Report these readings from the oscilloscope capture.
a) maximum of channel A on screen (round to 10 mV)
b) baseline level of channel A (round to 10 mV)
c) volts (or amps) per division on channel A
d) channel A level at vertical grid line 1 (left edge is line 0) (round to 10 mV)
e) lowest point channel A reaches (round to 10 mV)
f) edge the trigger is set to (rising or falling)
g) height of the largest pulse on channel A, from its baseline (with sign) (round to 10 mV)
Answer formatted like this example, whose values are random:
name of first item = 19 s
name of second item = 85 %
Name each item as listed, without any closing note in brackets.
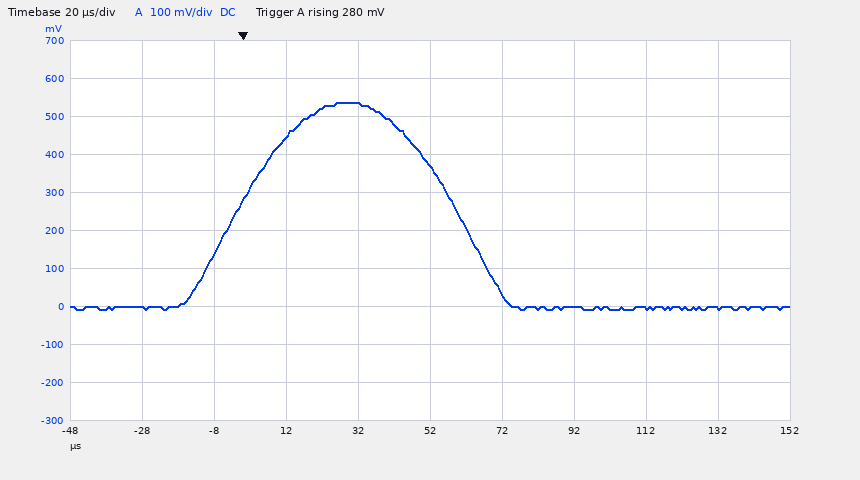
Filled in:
maximum of channel A on screen = 540 mV
baseline level of channel A = 0 mV
volts (or amps) per division on channel A = 100 mV
channel A level at vertical grid line 1 (left edge is line 0) = 0 mV
lowest point channel A reaches = -10 mV
edge the trigger is set to = rising
height of the largest pulse on channel A, from its baseline (with sign) = +540 mV
